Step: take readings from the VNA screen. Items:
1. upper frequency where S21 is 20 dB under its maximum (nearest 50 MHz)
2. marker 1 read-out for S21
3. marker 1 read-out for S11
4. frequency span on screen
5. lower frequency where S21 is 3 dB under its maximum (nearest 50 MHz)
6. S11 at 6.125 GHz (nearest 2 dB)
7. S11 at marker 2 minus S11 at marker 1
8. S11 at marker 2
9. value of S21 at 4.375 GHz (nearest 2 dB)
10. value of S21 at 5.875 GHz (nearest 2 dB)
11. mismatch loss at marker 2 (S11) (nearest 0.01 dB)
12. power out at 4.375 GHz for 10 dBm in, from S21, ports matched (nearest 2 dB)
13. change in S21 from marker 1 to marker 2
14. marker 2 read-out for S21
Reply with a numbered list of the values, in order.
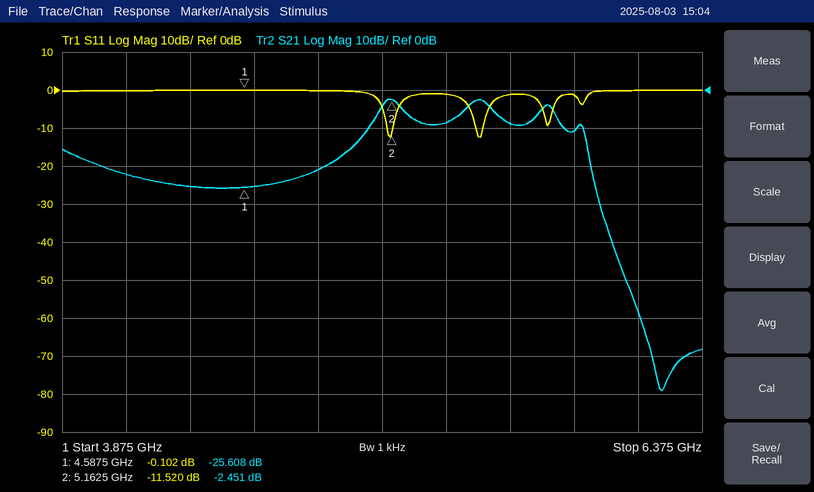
1. 5.95 GHz
2. -25.608 dB
3. -0.102 dB
4. 2.5 GHz
5. 5.10 GHz
6. 0 dB
7. -11.418 dB
8. -11.520 dB
9. -26 dB
10. -10 dB
11. 0.32 dB
12. -16 dBm
13. 23.157 dB
14. -2.451 dB
